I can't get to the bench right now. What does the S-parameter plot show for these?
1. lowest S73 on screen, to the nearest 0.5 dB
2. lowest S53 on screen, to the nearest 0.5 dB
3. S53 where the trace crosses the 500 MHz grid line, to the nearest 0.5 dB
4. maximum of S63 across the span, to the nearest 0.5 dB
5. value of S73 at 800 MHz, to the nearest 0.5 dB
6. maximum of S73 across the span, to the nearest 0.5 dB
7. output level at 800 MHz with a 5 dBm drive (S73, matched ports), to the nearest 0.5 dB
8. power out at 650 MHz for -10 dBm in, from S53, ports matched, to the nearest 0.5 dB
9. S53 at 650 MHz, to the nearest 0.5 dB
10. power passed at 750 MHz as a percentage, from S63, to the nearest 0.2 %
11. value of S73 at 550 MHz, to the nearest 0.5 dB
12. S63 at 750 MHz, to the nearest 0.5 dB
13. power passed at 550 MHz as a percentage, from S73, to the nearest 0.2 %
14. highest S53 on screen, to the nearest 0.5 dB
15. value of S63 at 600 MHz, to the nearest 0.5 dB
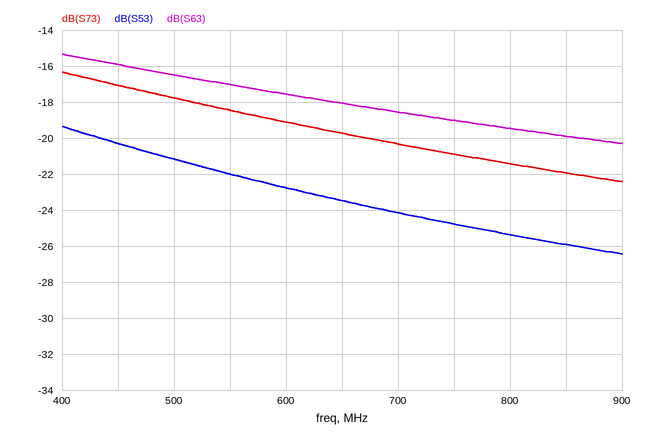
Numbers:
-22.5 dB
-26.5 dB
-21.0 dB
-15.5 dB
-21.5 dB
-16.5 dB
-16.5 dBm
-33.5 dBm
-23.5 dB
1.2 %
-18.5 dB
-19.0 dB
1.4 %
-19.5 dB
-17.5 dB
